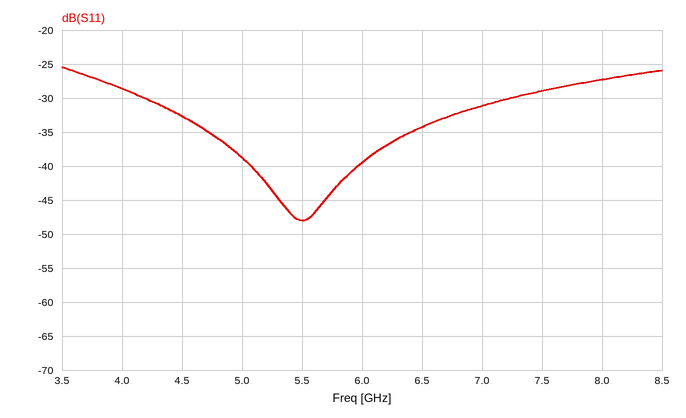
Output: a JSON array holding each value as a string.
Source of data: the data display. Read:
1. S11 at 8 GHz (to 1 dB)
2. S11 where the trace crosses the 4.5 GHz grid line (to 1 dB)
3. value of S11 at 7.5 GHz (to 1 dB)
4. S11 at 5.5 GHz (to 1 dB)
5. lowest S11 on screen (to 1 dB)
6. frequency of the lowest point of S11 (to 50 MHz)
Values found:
["-27 dB", "-33 dB", "-29 dB", "-48 dB", "-48 dB", "5.50 GHz"]
